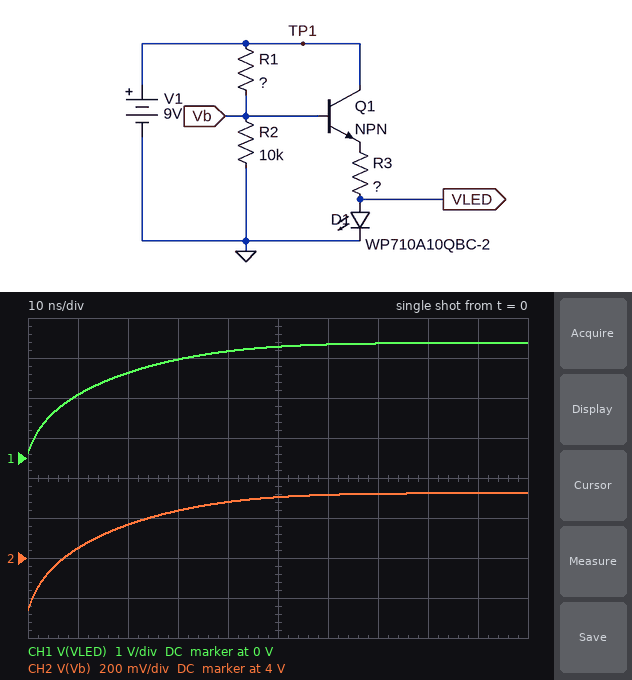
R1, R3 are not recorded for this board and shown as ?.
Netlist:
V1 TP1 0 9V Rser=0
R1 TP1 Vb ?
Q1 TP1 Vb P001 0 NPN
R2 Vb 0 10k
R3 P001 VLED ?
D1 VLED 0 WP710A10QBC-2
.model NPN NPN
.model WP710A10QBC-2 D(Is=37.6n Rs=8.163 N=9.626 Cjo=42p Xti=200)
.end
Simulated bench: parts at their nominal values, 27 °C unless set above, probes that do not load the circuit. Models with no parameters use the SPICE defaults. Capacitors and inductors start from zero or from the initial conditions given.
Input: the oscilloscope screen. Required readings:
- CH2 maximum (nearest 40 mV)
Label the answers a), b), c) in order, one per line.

a) 4.32 V
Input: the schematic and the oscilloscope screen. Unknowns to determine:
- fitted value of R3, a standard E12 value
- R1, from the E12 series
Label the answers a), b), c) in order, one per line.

a) 180 Ω
b) 10 kΩ
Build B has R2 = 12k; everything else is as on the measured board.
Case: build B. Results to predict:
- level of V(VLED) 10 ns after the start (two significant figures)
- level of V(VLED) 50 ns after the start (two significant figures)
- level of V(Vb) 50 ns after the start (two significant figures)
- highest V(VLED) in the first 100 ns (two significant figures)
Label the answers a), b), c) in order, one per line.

a) 1.7 V
b) 2.9 V
c) 4.6 V
d) 3.0 V
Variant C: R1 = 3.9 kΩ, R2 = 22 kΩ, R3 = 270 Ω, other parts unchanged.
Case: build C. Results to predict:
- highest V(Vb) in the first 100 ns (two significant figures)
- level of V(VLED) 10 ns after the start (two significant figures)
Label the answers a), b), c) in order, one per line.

a) 7.3 V
b) 2.1 V
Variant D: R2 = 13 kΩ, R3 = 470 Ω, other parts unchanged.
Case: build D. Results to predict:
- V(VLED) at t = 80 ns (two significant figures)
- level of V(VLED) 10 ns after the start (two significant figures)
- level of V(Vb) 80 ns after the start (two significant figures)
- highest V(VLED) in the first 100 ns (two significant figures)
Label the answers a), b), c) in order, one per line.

a) 2.7 V
b) 1.1 V
c) 4.9 V
d) 2.8 V
